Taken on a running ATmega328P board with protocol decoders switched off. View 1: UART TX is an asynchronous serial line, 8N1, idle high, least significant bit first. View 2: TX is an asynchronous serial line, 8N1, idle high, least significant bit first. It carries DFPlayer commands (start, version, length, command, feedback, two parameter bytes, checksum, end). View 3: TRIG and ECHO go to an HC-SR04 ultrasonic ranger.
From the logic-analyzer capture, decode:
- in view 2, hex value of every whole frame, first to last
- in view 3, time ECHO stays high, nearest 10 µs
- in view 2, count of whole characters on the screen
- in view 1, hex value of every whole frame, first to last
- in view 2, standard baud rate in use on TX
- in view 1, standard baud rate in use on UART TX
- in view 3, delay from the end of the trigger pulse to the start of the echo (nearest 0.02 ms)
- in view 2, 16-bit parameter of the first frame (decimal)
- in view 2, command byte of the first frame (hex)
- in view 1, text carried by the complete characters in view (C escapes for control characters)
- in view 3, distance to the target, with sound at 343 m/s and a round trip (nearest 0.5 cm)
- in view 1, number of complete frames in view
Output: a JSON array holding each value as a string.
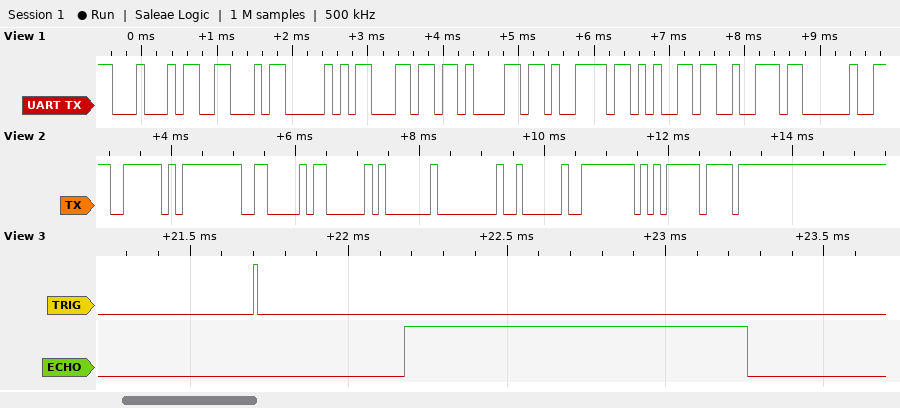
["7E FF 06 03 01 00 02 FE F5 EF", "1080 µs", "10", "44 46 50 6C 61 79 65 72 20", "9600 baud", "9600 baud", "0.46 ms", "2", "0x03", "\"DFPlayer \"", "18.5 cm", "9"]
